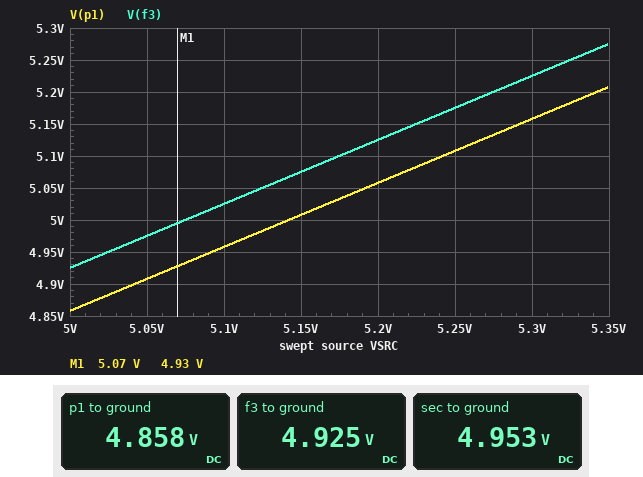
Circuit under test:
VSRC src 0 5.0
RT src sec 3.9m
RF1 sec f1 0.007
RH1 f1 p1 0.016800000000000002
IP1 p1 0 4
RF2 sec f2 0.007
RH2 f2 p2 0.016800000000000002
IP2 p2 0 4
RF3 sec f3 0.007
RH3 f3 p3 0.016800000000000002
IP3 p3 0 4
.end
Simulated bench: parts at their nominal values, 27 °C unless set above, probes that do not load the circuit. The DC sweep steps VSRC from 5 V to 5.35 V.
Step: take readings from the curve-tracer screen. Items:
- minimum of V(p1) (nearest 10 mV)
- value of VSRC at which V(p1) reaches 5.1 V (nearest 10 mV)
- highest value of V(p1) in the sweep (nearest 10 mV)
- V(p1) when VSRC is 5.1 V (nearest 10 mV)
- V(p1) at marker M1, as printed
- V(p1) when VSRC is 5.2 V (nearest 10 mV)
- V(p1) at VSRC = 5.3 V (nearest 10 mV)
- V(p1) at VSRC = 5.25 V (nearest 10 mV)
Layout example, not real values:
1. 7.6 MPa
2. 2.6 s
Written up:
1. 4.86 V
2. 5.24 V
3. 5.21 V
4. 4.96 V
5. 4.93 V
6. 5.06 V
7. 5.16 V
8. 5.11 V
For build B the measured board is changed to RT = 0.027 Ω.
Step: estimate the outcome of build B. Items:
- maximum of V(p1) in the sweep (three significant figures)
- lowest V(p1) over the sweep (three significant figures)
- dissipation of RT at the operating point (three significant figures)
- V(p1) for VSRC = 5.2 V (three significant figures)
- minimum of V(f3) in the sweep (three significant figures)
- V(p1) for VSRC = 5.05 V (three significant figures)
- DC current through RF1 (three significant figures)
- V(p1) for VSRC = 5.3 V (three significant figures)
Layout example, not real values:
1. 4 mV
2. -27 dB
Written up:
1. 4.93 V
2. 4.58 V
3. 3.89 W
4. 4.78 V
5. 4.65 V
6. 4.63 V
7. 4.00 A
8. 4.88 V
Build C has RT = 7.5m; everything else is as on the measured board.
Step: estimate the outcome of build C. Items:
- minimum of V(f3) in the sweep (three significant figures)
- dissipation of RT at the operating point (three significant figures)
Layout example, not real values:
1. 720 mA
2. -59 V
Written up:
1. 4.88 V
2. 1.08 W
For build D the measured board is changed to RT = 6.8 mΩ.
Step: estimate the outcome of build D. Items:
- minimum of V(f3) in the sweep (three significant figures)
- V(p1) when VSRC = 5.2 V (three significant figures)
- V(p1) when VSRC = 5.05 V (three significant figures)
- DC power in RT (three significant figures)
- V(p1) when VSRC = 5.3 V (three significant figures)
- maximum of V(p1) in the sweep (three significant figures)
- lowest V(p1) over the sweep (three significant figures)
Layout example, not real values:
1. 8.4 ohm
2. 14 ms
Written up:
1. 4.89 V
2. 5.02 V
3. 4.87 V
4. 979 mW
5. 5.12 V
6. 5.17 V
7. 4.82 V
